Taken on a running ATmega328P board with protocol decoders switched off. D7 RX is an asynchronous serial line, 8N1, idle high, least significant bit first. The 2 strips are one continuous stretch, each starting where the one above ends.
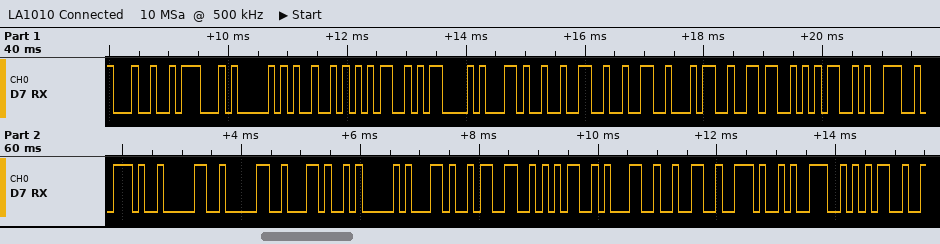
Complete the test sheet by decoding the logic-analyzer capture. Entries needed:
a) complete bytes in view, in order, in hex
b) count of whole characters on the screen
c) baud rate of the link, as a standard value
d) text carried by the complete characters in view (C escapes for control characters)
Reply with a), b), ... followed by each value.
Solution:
a) 24 47 50 52 4D 43 2C 32 32 34 36 35 39 2E 30 30 2C 41 2C 33 35 31 32 2E 39 35
b) 26
c) 9600 baud
d) "$GPRMC,224659.00,A,3512.95"
